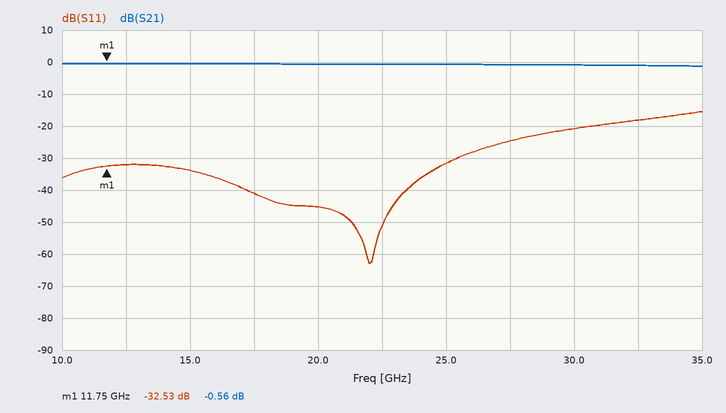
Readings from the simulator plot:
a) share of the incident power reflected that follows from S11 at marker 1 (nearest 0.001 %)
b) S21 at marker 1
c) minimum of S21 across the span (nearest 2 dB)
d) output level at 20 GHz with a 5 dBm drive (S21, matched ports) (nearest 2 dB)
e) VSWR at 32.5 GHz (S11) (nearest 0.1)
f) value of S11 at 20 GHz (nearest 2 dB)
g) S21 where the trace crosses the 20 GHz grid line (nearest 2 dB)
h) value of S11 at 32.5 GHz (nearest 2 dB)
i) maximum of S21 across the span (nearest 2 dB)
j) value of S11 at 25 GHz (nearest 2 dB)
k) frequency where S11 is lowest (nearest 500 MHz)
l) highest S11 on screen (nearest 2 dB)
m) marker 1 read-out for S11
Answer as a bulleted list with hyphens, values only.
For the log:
- 0.056 %
- -0.56 dB
- -2 dB
- 4 dBm
- 1.3
- -46 dB
- 0 dB
- -18 dB
- 0 dB
- -32 dB
- 22.0 GHz
- -16 dB
- -32.53 dB
